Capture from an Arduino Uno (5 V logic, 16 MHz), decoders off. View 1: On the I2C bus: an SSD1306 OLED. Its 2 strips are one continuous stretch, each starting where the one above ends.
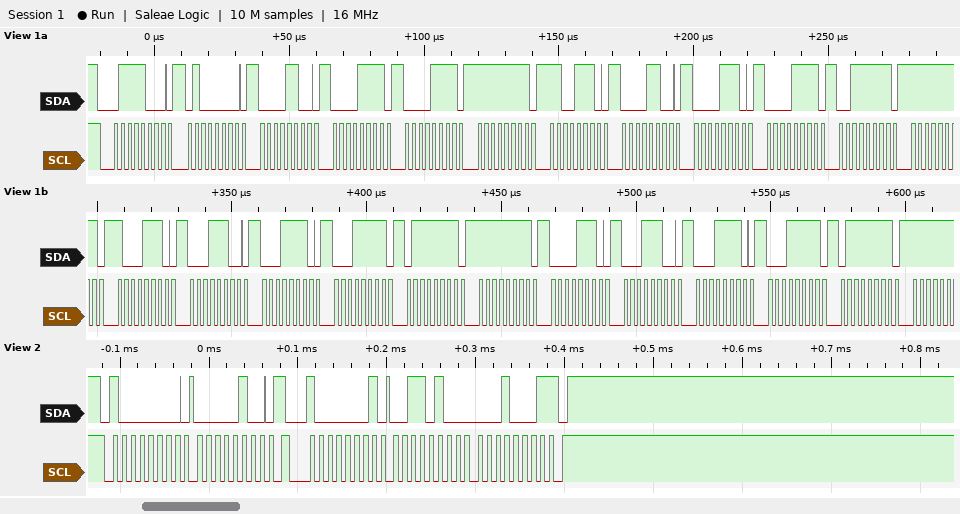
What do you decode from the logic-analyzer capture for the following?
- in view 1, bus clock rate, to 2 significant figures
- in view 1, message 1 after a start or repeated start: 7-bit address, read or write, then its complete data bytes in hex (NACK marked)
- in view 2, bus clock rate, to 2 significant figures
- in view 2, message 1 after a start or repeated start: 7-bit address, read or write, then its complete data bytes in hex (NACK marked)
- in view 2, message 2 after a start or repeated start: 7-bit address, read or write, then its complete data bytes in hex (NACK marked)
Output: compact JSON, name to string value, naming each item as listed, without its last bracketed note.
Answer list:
{"in view 1, bus clock rate, to 2 significant figures": "400 kHz", "in view 1, message 1 after a start or repeated start: 7-bit address, read or write, then its complete data bytes in hex": "0x3C write: 40 0C 0F 0F FF CE 0C 0E 0F 3F FF 8E 1C 1E 1F 7F FF 0E 1C 1E 1F 7F", "in view 2, bus clock rate, to 2 significant figures": "100 kHz", "in view 2, message 1 after a start or repeated start: 7-bit address, read or write, then its complete data bytes in hex": "0x40 write: 04", "in view 2, message 2 after a start or repeated start: 7-bit address, read or write, then its complete data bytes in hex": "0x40 read: 34 11 NACK"}
